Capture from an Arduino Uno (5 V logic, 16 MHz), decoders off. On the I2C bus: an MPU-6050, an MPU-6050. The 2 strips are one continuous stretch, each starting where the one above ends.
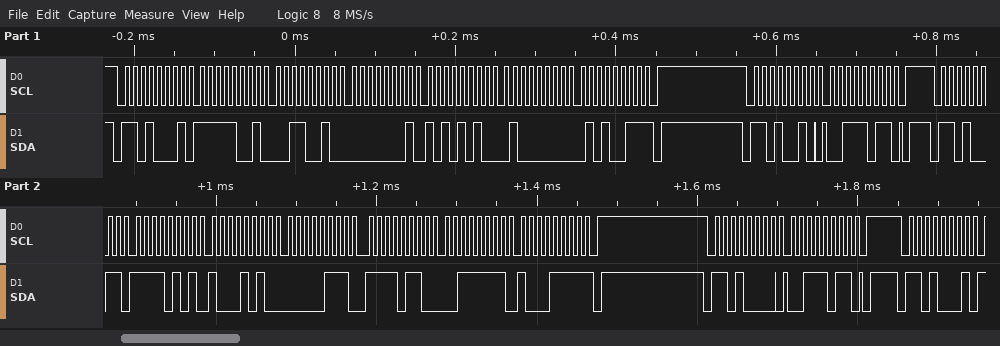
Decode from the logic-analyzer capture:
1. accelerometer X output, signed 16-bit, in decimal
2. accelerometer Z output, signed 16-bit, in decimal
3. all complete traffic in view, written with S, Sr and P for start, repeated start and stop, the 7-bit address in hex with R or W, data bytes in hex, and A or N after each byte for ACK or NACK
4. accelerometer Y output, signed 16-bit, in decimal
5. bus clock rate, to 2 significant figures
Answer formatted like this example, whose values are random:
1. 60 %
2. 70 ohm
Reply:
1. -2678
2. 16271
3. S 68R A F9 A 32 A 01 A AA A 40 A 53 N P S 69W A 3B A P S 69R A F5 A 8A A 07 A F6 A 3F A 8F N P S 68W A 3B A P S 68R A
4. 2038
5. 100 kHz
